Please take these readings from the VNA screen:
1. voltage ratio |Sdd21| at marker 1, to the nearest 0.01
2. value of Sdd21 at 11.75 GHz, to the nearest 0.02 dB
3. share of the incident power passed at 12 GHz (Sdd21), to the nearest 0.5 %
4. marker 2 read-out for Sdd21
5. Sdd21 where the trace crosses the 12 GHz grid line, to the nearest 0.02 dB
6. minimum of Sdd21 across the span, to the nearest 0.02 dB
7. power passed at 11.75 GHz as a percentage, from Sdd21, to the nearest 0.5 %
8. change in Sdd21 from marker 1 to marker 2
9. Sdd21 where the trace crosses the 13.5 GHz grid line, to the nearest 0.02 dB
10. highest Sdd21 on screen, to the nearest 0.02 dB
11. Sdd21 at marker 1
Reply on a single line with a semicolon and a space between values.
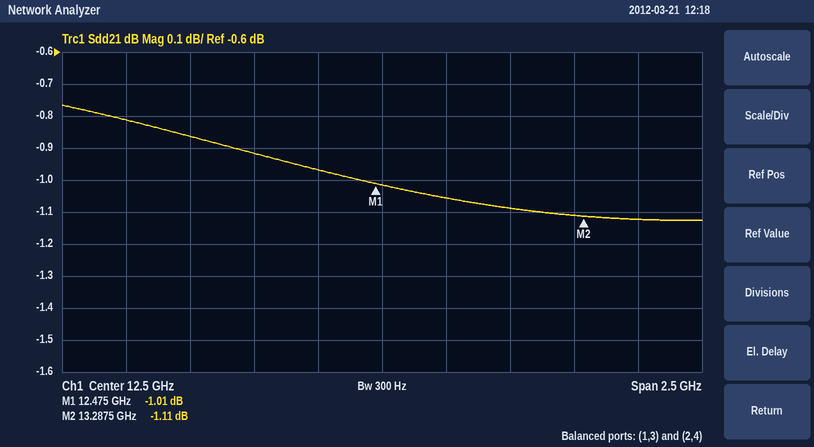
0.89; -0.86 dB; 81.0 %; -1.11 dB; -0.92 dB; -1.12 dB; 82.0 %; -0.10 dB; -1.12 dB; -0.76 dB; -1.01 dB
